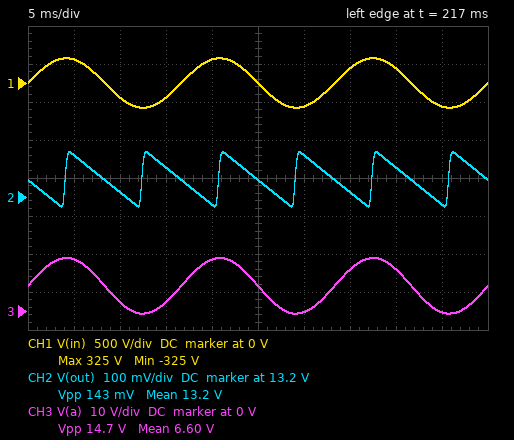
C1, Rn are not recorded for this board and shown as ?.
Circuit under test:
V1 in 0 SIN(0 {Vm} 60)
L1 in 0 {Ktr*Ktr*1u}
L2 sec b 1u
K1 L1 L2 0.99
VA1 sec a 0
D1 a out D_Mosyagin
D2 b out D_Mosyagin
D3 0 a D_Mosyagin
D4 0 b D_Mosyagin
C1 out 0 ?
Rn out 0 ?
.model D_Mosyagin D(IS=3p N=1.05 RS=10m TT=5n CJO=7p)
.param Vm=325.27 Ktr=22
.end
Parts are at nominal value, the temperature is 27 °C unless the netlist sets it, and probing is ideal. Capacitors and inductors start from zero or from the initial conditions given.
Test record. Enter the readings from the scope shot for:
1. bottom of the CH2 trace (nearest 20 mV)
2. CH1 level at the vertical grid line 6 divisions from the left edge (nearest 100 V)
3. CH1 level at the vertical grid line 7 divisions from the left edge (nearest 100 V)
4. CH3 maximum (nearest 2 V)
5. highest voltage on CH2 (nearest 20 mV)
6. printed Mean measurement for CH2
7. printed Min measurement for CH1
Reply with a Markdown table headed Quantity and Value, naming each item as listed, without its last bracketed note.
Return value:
| Quantity | Value |
|---|---|
| bottom of the CH2 trace | 13.18 V |
| CH1 level at the vertical grid line 6 divisions from the left edge | -300 V |
| CH1 level at the vertical grid line 7 divisions from the left edge | 200 V |
| CH3 maximum | 14 V |
| highest voltage on CH2 | 13.32 V |
| printed Mean measurement for CH2 | 13.2 V |
| printed Min measurement for CH1 | -325 V |
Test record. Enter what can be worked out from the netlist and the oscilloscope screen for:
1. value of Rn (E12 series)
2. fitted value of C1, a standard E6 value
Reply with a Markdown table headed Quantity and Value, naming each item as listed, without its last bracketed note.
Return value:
| Quantity | Value |
|---|---|
| value of Rn | 1 kΩ |
| fitted value of C1, a standard E6 value | 680 µF |
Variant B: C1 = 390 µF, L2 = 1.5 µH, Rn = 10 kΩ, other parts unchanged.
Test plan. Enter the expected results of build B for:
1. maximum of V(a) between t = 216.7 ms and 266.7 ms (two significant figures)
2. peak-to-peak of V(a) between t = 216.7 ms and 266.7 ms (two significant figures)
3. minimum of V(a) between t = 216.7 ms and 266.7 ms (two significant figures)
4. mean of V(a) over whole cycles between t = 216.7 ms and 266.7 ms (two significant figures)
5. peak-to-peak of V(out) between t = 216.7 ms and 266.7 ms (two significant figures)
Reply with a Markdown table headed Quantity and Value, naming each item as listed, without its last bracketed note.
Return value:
| Quantity | Value |
|---|---|
| maximum of V(a) between t = 216.7 ms and 266.7 ms | 17 V |
| peak-to-peak of V(a) between t = 216.7 ms and 266.7 ms | 18 V |
| minimum of V(a) between t = 216.7 ms and 266.7 ms | -630 mV |
| mean of V(a) over whole cycles between t = 216.7 ms and 266.7 ms | 8.3 V |
| peak-to-peak of V(out) between t = 216.7 ms and 266.7 ms | 32 mV |
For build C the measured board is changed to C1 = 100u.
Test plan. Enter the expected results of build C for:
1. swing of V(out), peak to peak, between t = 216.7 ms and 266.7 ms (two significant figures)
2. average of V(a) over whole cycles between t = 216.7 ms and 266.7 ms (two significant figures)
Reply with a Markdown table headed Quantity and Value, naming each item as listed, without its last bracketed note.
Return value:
| Quantity | Value |
|---|---|
| swing of V(out), peak to peak, between t = 216.7 ms and 266.7 ms | 910 mV |
| average of V(a) over whole cycles between t = 216.7 ms and 266.7 ms | 6.5 V |
